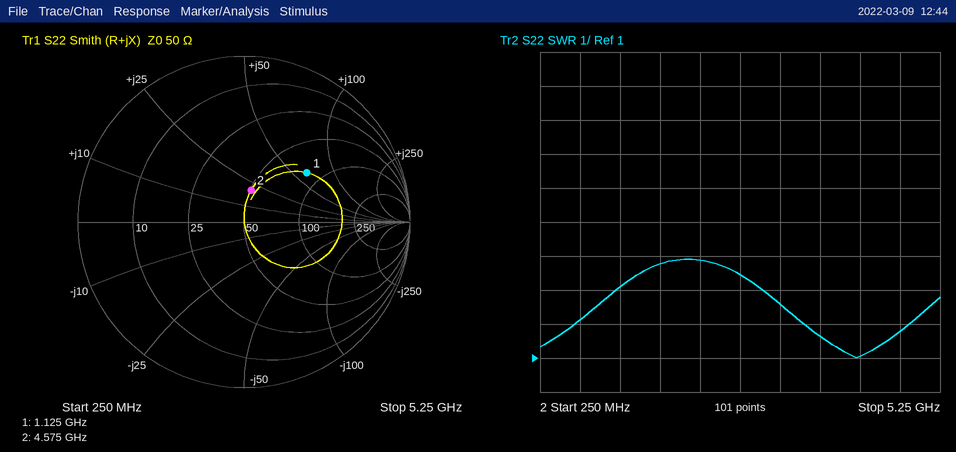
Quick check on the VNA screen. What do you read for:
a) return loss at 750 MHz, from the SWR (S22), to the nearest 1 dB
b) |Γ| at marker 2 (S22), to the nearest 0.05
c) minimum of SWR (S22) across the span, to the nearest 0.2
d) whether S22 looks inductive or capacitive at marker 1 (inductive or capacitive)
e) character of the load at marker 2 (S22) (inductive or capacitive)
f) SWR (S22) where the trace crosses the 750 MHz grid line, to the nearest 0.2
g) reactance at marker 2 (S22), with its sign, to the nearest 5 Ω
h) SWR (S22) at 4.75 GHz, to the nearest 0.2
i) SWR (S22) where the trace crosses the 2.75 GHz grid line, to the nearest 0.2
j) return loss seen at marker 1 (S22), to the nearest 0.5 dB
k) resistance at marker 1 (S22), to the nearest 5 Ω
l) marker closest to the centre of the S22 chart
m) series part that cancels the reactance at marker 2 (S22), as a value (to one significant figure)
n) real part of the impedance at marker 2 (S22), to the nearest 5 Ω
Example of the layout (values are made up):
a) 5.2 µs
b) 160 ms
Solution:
a) 9 dB
b) 0.20
c) 1.0
d) inductive
e) inductive
f) 2.2
g) +20 Ω
h) 1.8
i) 3.4
j) 6.5 dB
k) 80 Ω
l) marker 2
m) 2 pF
n) 50 Ω
